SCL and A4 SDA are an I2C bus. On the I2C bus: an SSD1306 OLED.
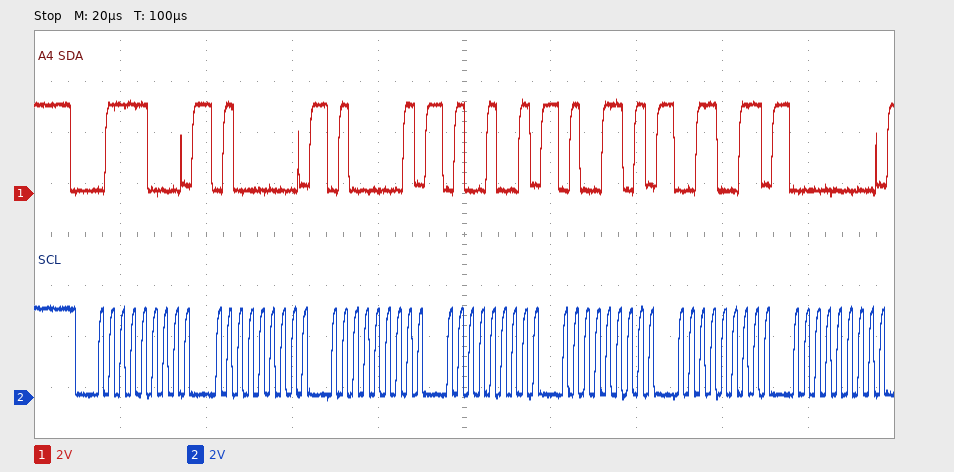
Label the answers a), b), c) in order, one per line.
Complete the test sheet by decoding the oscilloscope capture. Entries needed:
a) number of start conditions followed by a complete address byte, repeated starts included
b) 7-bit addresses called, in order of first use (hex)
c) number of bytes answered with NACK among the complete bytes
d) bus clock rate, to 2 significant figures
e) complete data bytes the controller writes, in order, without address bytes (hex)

a) 1
b) 0x3C
c) 0
d) 400 kHz
e) 40 41 49 4D 33 00
